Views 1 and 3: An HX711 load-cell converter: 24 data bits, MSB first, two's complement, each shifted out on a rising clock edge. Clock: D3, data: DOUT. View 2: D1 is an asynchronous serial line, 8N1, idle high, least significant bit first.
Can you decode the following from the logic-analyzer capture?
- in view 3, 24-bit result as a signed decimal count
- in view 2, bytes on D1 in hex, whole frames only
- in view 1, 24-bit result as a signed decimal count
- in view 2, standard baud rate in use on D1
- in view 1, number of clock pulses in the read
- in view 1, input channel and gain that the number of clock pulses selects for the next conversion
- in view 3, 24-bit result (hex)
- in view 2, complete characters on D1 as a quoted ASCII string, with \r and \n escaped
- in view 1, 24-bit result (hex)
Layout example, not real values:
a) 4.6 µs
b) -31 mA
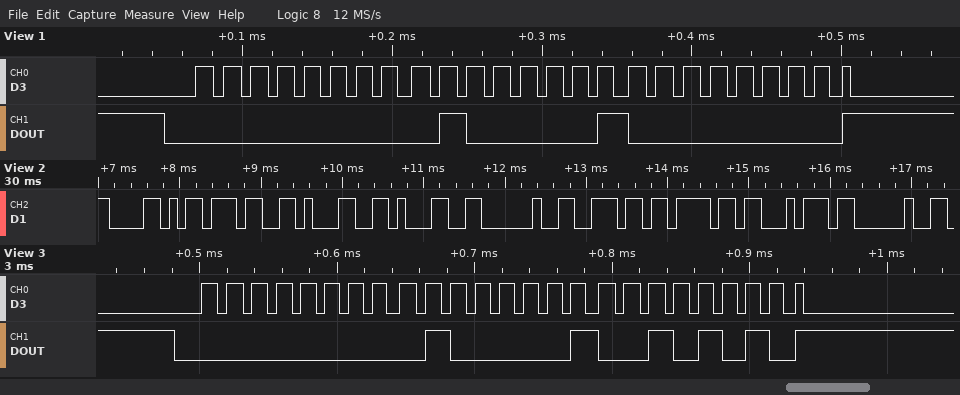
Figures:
a) 16682
b) 58 37 31 31 20 6E 6F 74 20
c) 16640
d) 9600 baud
e) 25
f) channel A, gain 128
g) 0x00412A
h) "X711 not "
i) 0x004100
